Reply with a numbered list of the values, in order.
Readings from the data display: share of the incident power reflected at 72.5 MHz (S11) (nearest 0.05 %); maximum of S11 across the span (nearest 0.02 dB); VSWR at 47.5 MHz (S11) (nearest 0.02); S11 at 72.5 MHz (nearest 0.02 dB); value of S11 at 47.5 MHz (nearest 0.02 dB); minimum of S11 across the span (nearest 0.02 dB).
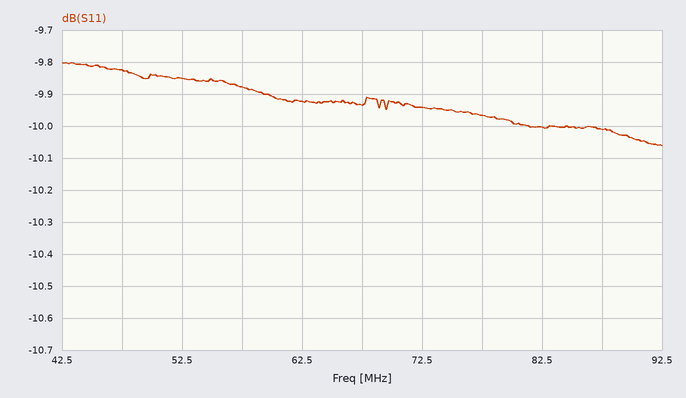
1. 10.15 %
2. -9.80 dB
3. 1.96
4. -9.94 dB
5. -9.82 dB
6. -10.06 dB
